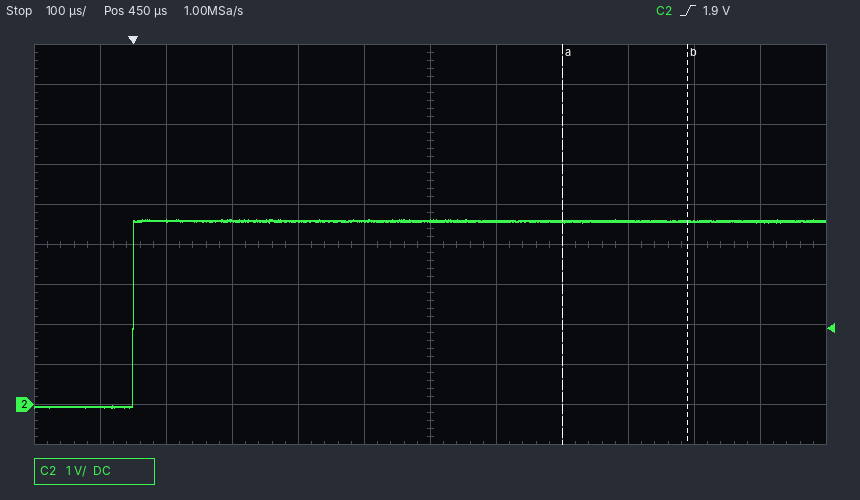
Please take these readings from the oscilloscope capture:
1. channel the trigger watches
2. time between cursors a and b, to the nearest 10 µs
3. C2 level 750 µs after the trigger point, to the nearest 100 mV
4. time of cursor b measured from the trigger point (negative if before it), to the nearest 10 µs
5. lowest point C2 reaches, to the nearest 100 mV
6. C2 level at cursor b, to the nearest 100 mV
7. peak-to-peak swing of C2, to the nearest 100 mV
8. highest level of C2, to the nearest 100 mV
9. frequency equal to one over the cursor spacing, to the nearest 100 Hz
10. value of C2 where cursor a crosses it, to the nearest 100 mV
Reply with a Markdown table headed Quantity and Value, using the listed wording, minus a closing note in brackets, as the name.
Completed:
| Quantity | Value |
|---|---|
| channel the trigger watches | C2 |
| time between cursors a and b, to the nearest 10 µs | 190 µs |
| C2 level 750 µs after the trigger point, to the nearest 100 mV | 4.6 V |
| time of cursor b measured from the trigger point (negative if before it), to the nearest 10 µs | +840 µs |
| lowest point C2 reaches, to the nearest 100 mV | -100 mV |
| C2 level at cursor b, to the nearest 100 mV | 4.6 V |
| peak-to-peak swing of C2, to the nearest 100 mV | 4.7 V |
| highest level of C2, to the nearest 100 mV | 4.6 V |
| frequency equal to one over the cursor spacing, to the nearest 100 Hz | 5.3 kHz |
| value of C2 where cursor a crosses it, to the nearest 100 mV | 4.6 V |
